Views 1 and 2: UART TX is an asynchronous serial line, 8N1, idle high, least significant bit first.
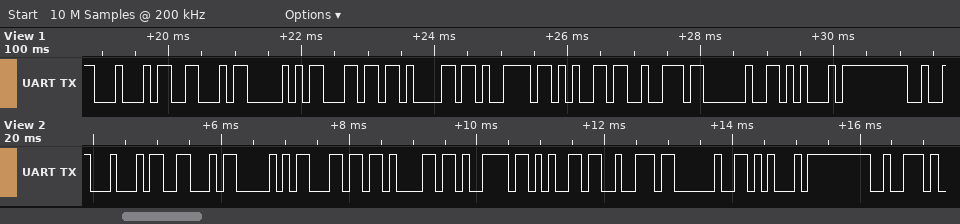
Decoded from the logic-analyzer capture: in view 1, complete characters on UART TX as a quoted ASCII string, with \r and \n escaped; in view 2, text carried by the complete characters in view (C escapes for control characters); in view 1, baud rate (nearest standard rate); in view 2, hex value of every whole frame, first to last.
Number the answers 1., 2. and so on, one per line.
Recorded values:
1. "DFPlayer E"
2. "DFPlayer Er"
3. 9600 baud
4. 44 46 50 6C 61 79 65 72 20 45 72
